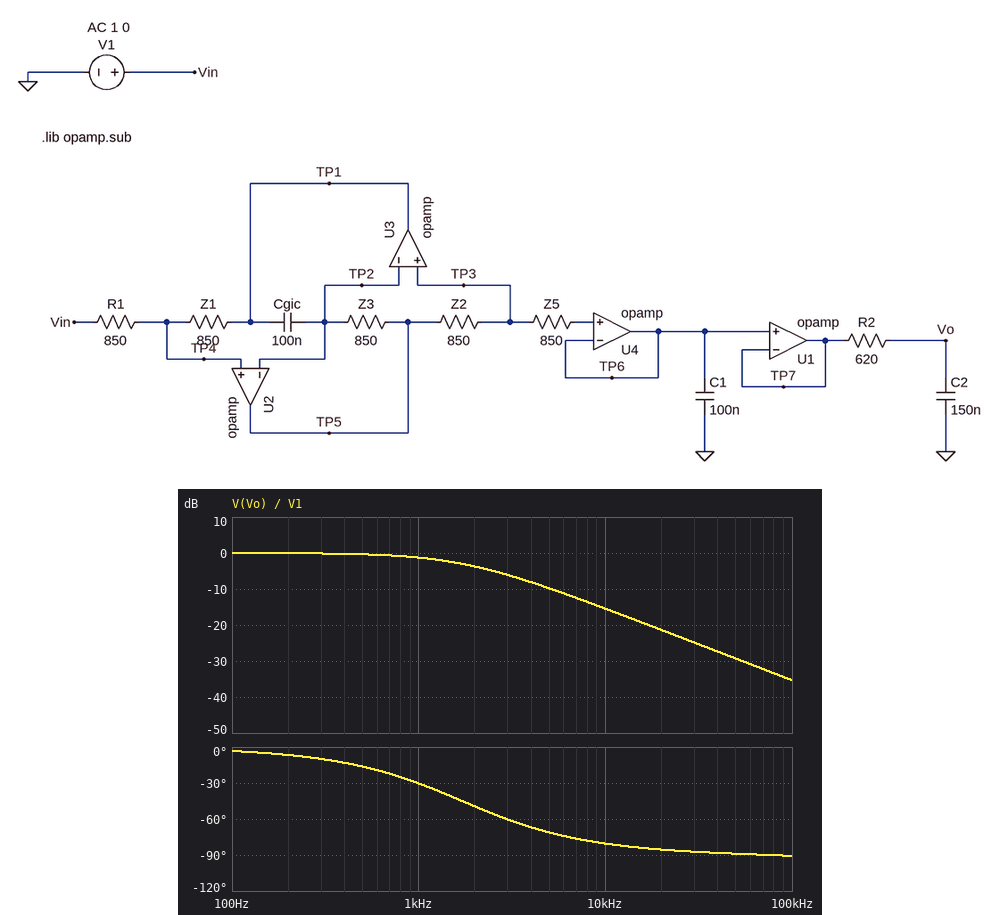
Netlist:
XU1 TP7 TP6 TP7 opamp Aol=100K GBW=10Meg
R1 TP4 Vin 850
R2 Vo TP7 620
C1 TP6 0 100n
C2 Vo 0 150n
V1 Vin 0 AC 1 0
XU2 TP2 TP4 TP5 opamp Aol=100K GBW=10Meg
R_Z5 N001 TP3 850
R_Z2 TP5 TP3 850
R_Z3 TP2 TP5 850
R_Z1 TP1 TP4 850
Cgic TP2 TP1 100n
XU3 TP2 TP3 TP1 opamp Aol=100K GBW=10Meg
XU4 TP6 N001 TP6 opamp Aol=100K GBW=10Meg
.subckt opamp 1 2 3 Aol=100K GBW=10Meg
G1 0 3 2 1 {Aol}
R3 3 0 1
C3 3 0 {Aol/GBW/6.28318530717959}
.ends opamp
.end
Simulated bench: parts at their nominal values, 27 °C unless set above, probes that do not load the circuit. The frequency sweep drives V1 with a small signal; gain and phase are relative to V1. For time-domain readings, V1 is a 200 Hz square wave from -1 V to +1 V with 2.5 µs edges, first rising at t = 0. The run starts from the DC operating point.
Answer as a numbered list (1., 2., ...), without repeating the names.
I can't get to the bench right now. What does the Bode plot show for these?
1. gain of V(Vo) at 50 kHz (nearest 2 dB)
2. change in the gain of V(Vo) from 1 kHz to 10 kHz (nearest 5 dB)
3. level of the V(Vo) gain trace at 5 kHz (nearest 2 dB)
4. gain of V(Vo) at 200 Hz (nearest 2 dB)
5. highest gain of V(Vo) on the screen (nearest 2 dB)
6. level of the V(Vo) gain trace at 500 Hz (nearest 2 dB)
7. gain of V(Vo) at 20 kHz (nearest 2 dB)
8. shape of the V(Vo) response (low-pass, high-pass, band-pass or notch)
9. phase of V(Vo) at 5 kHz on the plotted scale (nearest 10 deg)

1. -30 dB
2. -15 dB
3. -10 dB
4. 0 dB
5. 0 dB
6. 0 dB
7. -22 dB
8. low-pass
9. -70 deg
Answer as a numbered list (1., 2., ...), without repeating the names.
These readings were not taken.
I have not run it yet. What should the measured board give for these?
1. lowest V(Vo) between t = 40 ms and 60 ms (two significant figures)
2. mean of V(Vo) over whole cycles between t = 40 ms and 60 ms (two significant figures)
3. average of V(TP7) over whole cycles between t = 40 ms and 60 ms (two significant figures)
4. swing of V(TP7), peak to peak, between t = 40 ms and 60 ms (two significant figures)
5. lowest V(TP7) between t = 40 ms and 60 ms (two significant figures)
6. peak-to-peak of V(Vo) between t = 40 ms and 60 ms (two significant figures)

1. -510 mV
2. 490 mV
3. 490 mV
4. 2.0 V
5. -510 mV
6. 2.0 V
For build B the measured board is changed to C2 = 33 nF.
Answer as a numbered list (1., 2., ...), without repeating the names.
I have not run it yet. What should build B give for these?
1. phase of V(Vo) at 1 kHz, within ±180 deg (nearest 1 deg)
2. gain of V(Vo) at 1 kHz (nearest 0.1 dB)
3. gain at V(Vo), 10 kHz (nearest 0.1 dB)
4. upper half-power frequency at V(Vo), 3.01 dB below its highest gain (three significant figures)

1. -7 deg
2. -0.1 dB
3. -4.2 dB
4. 7.78 kHz
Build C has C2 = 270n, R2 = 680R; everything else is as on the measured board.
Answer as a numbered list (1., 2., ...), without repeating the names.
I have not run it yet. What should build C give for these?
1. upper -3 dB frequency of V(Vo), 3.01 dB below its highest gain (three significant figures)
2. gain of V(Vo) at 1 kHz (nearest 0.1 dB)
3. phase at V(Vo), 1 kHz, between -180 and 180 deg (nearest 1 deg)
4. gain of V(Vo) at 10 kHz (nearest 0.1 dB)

1. 867 Hz
2. -3.7 dB
3. -49 deg
4. -21.3 dB
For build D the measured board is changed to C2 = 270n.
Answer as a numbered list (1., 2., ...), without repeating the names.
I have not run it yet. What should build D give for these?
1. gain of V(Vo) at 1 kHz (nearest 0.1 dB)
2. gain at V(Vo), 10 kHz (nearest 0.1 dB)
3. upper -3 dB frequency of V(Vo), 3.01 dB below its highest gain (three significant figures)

1. -3.2 dB
2. -20.5 dB
3. 951 Hz
